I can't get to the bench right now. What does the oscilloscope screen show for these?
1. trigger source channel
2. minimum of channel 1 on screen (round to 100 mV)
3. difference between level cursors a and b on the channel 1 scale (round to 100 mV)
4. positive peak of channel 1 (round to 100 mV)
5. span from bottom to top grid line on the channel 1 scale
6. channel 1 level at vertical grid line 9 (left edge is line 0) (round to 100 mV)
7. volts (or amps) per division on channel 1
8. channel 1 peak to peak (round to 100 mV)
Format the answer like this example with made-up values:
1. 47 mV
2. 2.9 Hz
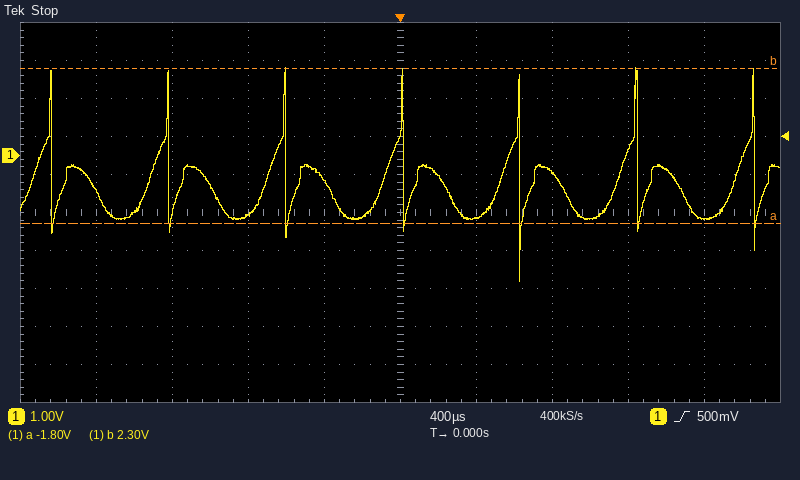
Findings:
1. channel 1
2. -3.3 V
3. 4.1 V
4. 2.3 V
5. 10 V
6. -1.7 V
7. 1 V
8. 5.6 V
